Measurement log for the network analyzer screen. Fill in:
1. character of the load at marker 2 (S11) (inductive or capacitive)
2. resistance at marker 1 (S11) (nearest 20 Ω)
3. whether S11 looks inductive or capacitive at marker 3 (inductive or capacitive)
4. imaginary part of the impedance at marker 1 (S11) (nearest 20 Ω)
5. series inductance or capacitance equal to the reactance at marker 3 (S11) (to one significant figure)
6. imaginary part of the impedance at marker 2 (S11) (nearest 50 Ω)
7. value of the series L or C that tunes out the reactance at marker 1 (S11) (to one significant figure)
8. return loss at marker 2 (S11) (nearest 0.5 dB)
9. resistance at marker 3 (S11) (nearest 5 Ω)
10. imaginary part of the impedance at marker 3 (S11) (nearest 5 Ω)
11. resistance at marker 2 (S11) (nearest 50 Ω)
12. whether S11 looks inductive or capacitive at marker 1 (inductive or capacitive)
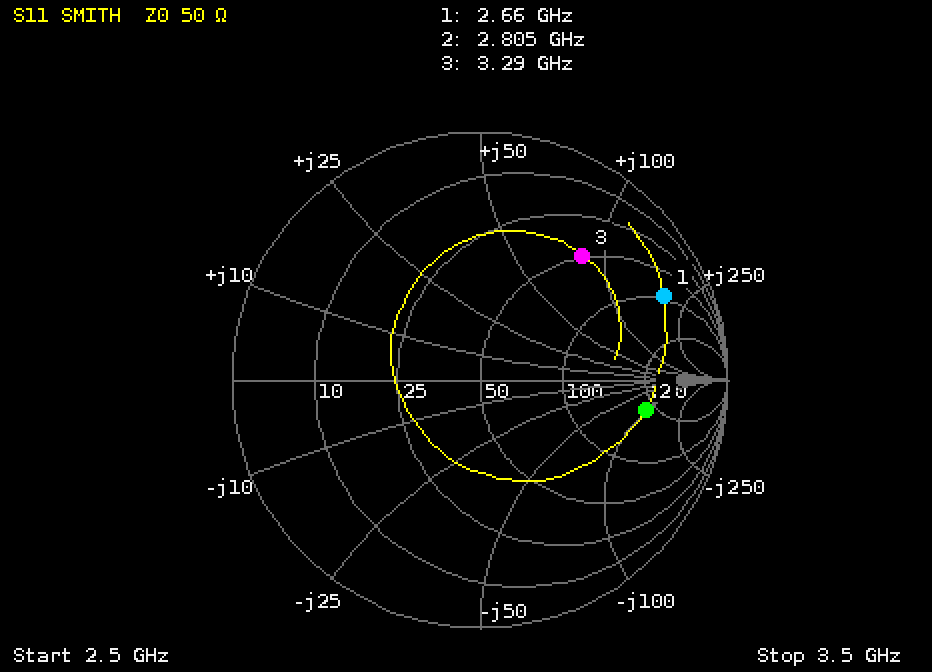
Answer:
capacitive
100 Ω
inductive
+180 Ω
4 nH
-100 Ω
300 fF
3.5 dB
50 Ω
+85 Ω
200 Ω
inductive
